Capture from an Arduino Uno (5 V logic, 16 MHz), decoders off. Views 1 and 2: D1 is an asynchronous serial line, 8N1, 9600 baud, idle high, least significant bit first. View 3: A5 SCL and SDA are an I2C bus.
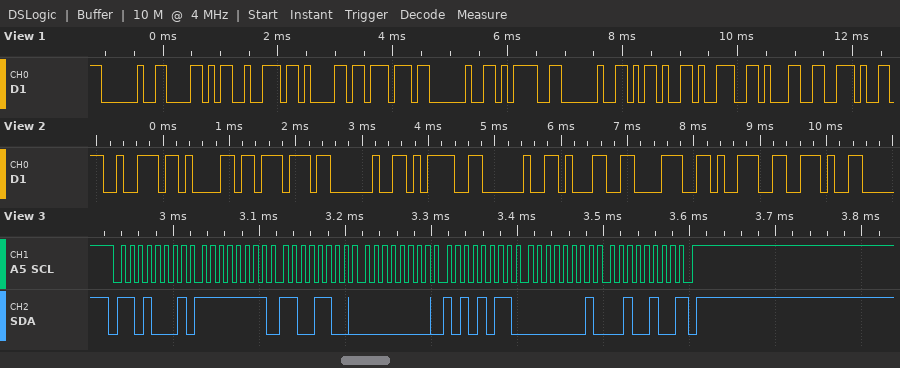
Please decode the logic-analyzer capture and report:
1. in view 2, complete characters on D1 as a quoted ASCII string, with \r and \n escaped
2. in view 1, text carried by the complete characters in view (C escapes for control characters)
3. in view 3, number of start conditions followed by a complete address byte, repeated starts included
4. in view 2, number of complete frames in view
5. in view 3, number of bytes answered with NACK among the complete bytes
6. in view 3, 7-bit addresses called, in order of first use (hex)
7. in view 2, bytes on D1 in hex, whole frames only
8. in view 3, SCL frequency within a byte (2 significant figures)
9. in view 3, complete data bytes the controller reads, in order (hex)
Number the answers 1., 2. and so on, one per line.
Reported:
1. "raw = 189."
2. " Xraw = -91."
3. 1
4. 10
5. 1
6. 0x68
7. 72 61 77 20 3D 20 31 38 39 2E
8. 100 kHz
9. FF CC 00 AB 01 24
